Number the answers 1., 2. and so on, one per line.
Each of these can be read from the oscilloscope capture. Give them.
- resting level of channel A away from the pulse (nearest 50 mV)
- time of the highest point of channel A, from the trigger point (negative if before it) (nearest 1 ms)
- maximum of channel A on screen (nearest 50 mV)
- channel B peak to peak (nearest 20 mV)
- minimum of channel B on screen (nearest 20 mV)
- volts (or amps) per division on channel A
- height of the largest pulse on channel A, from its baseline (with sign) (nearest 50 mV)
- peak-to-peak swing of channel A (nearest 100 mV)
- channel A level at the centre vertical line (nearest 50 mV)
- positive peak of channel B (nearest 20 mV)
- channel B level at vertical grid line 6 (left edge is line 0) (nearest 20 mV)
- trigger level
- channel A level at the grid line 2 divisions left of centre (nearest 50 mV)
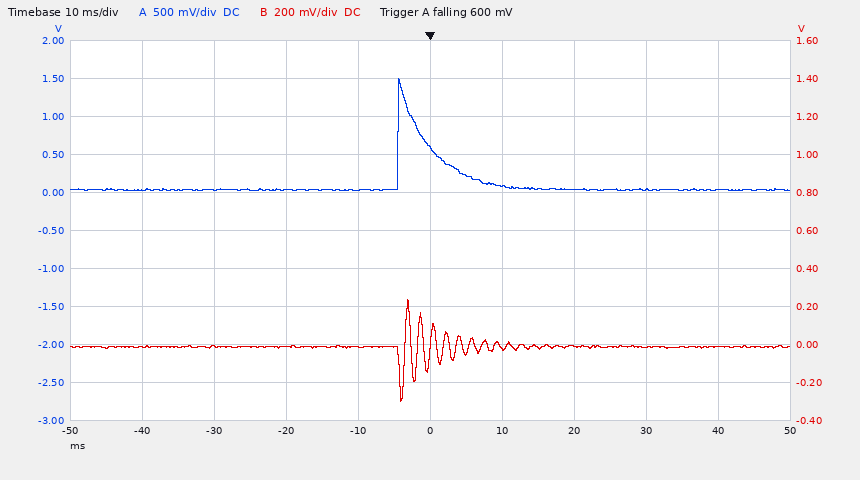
1. 50 mV
2. -4 ms
3. 1.50 V
4. 540 mV
5. -300 mV
6. 500 mV
7. +1.45 V
8. 1.50 V
9. 600 mV
10. 240 mV
11. -20 mV
12. 600 mV
13. 50 mV
